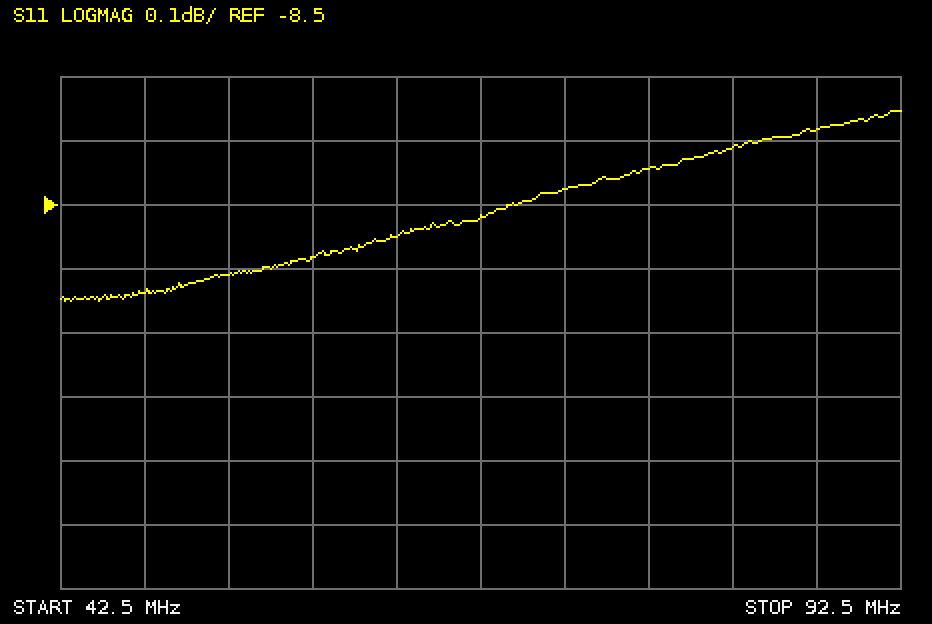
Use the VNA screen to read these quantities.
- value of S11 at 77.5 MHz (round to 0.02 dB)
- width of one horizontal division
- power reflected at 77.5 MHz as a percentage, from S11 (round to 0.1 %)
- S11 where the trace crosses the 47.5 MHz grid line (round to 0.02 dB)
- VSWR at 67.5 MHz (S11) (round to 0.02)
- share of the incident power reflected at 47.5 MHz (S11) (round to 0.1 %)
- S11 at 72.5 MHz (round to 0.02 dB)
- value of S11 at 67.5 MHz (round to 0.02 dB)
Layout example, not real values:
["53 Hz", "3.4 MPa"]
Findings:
["-8.44 dB", "5 MHz", "14.3 %", "-8.64 dB", "2.20", "13.7 %", "-8.48 dB", "-8.52 dB"]
